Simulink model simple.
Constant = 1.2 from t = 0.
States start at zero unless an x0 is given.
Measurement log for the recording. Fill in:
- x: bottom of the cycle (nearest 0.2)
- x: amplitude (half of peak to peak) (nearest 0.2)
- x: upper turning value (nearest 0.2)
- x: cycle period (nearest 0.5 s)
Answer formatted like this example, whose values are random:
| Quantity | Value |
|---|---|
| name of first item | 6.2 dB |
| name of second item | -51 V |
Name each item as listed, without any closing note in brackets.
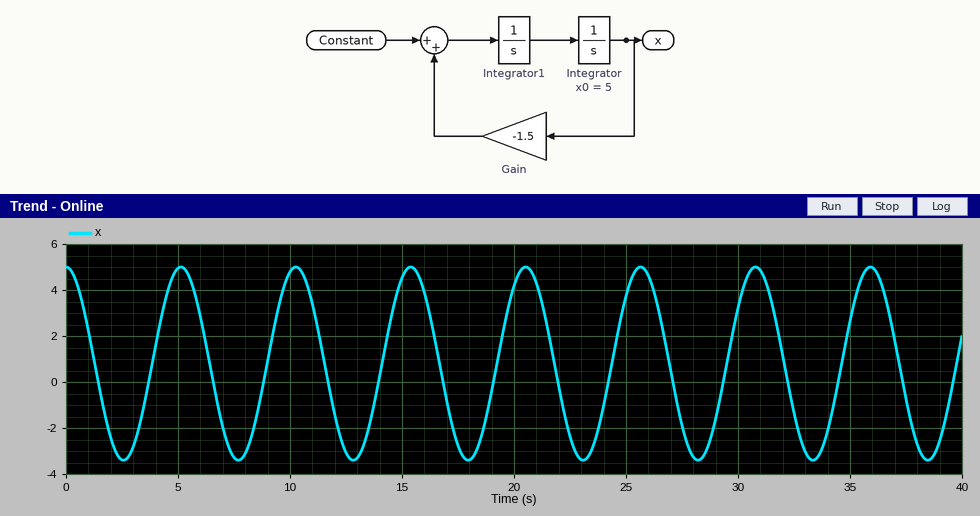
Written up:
| Quantity | Value |
|---|---|
| x: bottom of the cycle | -3.4 |
| x: amplitude (half of peak to peak) | 4.2 |
| x: upper turning value | 5.0 |
| x: cycle period | 5.0 s |
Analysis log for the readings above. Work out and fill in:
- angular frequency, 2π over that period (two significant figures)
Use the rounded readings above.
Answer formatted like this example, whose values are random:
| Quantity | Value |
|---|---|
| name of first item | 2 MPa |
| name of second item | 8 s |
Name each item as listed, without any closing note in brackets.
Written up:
| Quantity | Value |
|---|---|
| angular frequency, 2π over that period | 1.3 rad/s |
